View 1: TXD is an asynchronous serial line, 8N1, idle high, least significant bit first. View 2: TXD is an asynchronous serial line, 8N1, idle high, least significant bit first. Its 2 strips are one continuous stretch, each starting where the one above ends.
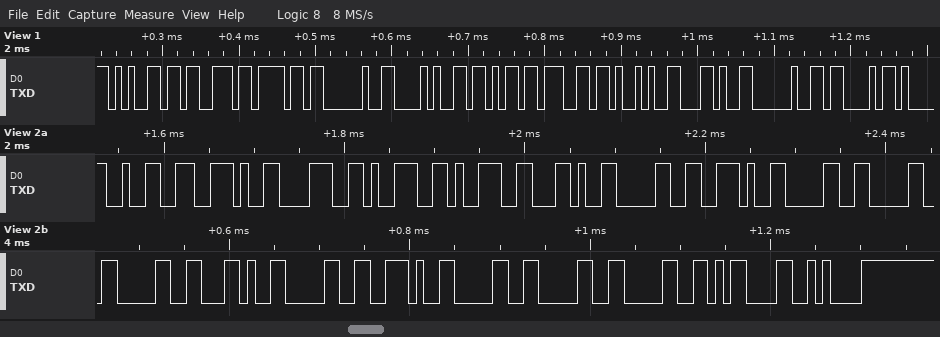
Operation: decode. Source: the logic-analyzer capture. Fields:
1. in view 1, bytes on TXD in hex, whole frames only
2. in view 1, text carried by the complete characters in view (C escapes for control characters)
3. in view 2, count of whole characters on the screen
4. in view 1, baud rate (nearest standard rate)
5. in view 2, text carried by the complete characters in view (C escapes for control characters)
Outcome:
65 73 6F 20 28 6B 67 29 2C 20 43
"eso (kg), C"
19
115200 baud
"2.899,0.000,0.000\r\n"
